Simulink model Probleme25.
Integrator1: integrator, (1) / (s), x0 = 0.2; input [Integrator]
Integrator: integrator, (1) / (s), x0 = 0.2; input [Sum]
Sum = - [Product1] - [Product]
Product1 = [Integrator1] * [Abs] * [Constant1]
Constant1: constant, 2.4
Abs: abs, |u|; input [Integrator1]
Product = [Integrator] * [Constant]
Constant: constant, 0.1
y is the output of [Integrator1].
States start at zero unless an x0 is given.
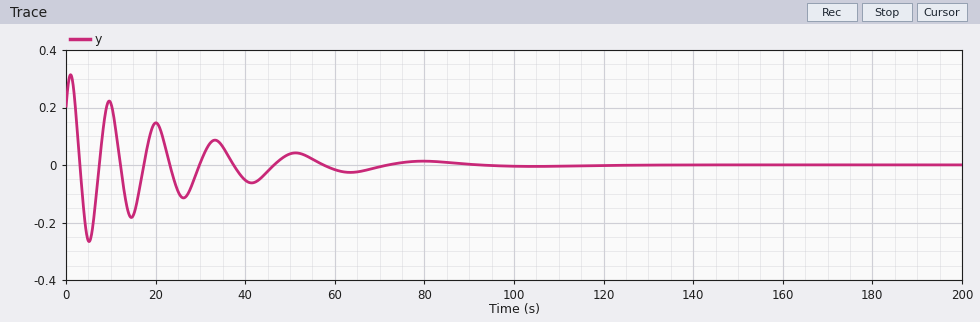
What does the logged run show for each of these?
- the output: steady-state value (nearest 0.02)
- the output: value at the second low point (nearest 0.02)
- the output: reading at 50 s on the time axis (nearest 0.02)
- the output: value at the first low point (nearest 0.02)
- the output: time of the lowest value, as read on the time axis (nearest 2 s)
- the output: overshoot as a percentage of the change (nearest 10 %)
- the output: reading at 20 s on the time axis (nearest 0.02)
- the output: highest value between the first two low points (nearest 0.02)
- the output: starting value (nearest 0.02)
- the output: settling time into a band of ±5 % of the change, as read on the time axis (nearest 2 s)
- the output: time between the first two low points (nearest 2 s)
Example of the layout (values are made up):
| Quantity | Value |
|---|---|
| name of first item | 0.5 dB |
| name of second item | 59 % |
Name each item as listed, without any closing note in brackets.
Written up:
| Quantity | Value |
|---|---|
| the output: steady-state value | 0.00 |
| the output: value at the second low point | -0.18 |
| the output: reading at 50 s on the time axis | 0.04 |
| the output: value at the first low point | -0.26 |
| the output: time of the lowest value, as read on the time axis | 6 s |
| the output: overshoot as a percentage of the change | 130 % |
| the output: reading at 20 s on the time axis | 0.14 |
| the output: highest value between the first two low points | 0.22 |
| the output: starting value | 0.20 |
| the output: settling time into a band of ±5 % of the change, as read on the time axis | 84 s |
| the output: time between the first two low points | 10 s |
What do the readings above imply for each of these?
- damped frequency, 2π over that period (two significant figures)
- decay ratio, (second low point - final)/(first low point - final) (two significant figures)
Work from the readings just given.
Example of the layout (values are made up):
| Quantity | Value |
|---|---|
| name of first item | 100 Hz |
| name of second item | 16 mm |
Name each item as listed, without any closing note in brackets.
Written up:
| Quantity | Value |
|---|---|
| damped frequency, 2π over that period | 0.63 rad/s |
| decay ratio, (second low point - final)/(first low point - final) | 0.69 |
